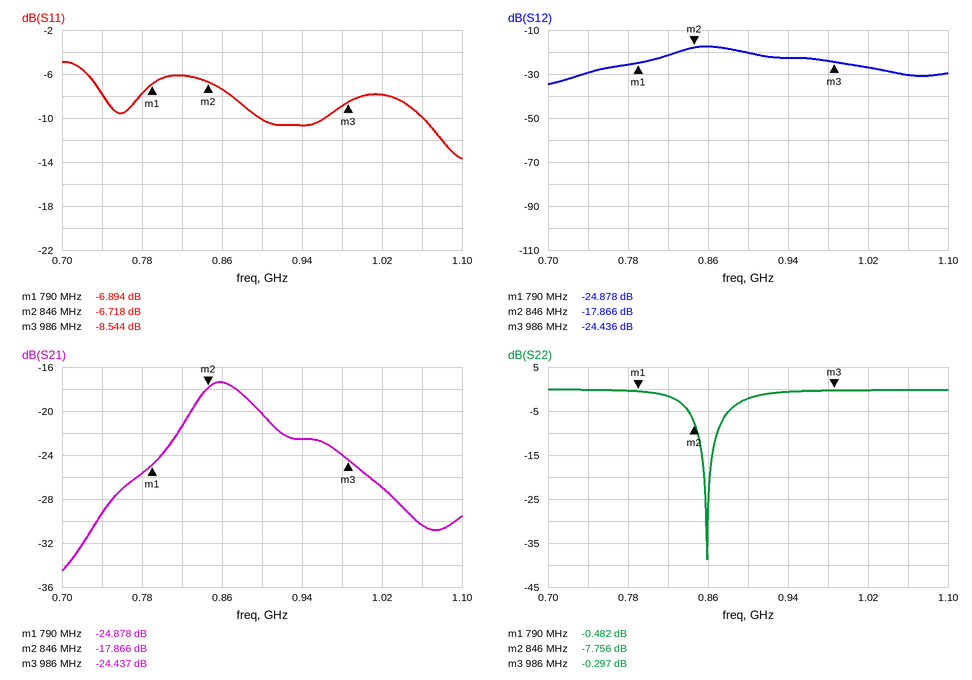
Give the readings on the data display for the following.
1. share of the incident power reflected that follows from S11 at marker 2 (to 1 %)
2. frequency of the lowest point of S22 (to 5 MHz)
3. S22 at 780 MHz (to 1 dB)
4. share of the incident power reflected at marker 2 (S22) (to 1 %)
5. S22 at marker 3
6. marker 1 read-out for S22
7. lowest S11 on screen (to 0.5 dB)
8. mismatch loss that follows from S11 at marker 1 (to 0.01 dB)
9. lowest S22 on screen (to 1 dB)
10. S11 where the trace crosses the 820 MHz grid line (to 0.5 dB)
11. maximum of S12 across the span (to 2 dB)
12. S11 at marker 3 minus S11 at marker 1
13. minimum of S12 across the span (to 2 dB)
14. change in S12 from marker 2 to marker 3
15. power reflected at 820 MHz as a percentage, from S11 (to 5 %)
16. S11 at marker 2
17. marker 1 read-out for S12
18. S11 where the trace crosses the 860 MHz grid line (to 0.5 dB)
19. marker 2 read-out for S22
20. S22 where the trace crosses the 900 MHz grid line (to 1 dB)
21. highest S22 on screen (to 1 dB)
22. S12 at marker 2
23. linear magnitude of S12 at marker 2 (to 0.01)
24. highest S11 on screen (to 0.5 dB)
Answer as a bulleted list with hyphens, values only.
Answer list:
- 21 %
- 860 MHz
- 0 dB
- 17 %
- -0.297 dB
- -0.482 dB
- -13.5 dB
- 0.99 dB
- -39 dB
- -6.0 dB
- -18 dB
- -1.650 dB
- -34 dB
- -6.570 dB
- 25 %
- -6.718 dB
- -24.878 dB
- -7.5 dB
- -7.756 dB
- -2 dB
- 0 dB
- -17.866 dB
- 0.13
- -5.0 dB
